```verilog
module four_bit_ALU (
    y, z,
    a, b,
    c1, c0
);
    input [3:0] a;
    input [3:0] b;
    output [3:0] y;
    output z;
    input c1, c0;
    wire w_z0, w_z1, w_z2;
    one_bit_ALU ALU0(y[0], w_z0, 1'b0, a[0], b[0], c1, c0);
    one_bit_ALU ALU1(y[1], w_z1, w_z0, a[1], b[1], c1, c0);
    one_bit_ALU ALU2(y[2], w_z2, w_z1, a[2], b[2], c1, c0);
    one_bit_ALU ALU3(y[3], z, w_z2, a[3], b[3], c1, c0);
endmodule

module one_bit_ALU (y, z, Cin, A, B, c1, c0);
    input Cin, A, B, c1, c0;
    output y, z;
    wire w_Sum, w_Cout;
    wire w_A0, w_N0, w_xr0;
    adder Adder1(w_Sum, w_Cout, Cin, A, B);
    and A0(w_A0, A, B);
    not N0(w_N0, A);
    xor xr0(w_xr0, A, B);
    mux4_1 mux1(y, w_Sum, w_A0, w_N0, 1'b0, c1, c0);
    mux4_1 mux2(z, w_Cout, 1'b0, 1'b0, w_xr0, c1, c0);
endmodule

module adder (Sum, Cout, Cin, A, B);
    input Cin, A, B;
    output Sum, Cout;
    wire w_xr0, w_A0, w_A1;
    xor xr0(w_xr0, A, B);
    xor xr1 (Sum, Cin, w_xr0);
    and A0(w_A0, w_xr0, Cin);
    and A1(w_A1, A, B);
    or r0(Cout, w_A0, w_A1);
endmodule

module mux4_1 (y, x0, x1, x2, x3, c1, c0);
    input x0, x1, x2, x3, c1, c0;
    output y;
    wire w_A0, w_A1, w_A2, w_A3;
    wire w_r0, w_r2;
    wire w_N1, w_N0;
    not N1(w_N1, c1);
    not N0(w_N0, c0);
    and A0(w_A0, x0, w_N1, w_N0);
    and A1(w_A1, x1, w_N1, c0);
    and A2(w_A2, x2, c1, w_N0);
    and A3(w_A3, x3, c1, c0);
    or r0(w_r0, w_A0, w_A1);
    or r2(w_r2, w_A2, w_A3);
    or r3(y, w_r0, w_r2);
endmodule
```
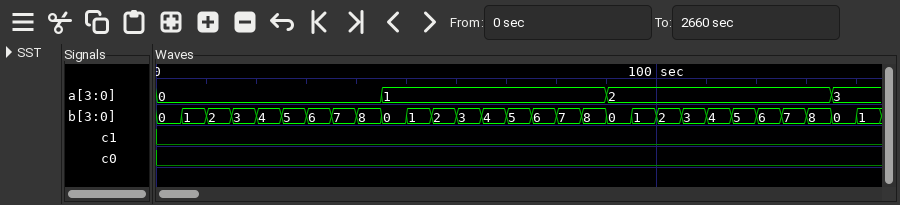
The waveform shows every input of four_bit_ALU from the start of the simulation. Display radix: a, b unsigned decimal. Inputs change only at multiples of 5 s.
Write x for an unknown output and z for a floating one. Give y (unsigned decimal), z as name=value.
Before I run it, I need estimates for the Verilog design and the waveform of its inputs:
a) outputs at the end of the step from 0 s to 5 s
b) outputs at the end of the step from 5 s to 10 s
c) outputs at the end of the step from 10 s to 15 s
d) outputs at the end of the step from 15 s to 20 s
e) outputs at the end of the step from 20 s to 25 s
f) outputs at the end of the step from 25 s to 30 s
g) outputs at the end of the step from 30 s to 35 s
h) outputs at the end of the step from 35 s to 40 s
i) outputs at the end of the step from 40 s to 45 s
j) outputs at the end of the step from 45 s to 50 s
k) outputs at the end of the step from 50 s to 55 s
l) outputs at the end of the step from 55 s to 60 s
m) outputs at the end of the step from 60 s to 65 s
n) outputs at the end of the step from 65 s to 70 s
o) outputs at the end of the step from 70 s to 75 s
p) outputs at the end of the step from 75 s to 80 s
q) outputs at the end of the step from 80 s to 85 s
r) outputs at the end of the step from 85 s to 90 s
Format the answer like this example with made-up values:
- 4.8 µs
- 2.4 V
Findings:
- y=0, z=0
- y=1, z=0
- y=2, z=0
- y=3, z=0
- y=4, z=0
- y=5, z=0
- y=6, z=0
- y=7, z=0
- y=8, z=0
- y=1, z=0
- y=2, z=0
- y=3, z=0
- y=4, z=0
- y=5, z=0
- y=6, z=0
- y=7, z=0
- y=8, z=0
- y=9, z=0
